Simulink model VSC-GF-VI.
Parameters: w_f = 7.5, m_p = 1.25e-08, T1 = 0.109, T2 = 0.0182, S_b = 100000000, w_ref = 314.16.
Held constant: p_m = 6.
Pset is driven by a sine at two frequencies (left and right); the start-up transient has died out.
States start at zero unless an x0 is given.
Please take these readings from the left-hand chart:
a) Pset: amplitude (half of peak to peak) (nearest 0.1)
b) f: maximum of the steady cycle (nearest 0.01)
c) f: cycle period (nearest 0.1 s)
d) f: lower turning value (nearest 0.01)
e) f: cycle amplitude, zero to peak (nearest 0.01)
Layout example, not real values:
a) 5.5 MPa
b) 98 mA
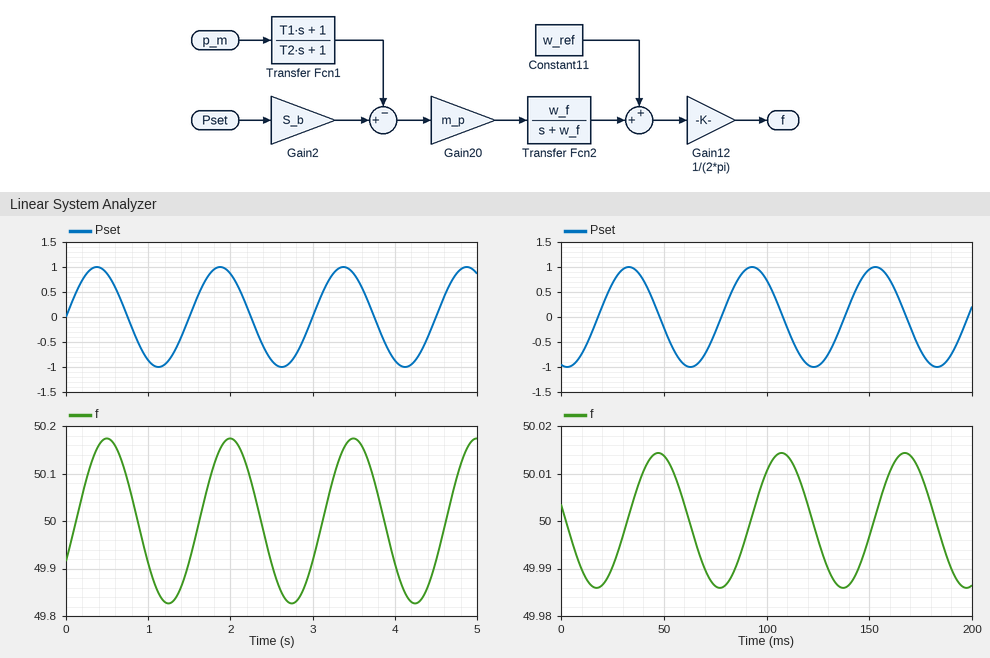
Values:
a) 1.0
b) 50.17
c) 1.5 s
d) 49.83
e) 0.17
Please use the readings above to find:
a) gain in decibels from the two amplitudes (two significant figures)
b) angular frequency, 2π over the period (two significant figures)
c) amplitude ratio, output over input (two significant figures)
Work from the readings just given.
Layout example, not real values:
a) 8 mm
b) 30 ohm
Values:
a) -15 dB
b) 4.2 rad/s
c) 0.17
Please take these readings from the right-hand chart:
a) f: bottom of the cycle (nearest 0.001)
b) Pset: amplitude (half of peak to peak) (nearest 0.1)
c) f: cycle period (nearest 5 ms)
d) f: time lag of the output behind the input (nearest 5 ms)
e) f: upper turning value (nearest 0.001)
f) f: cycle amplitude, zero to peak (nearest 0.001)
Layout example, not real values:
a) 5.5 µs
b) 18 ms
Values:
a) 49.986
b) 1.0
c) 60 ms
d) 15 ms
e) 50.014
f) 0.014
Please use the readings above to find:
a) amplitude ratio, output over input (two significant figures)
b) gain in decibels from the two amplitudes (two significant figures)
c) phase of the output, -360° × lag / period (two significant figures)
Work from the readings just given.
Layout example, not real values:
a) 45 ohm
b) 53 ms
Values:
a) 0.014
b) -37 dB
c) -90°
